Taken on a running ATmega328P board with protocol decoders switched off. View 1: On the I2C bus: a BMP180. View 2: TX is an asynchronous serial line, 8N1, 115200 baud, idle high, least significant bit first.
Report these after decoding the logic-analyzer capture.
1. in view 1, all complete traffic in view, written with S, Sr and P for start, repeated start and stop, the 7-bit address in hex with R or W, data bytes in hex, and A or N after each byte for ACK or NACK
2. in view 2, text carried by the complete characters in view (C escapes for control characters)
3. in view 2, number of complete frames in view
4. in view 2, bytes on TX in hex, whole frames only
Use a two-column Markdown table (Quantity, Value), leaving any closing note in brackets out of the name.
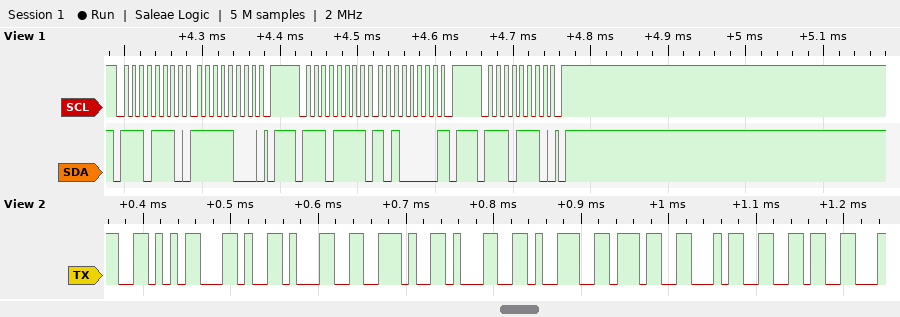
| Quantity | Value |
|---|---|
| in view 1, all complete traffic in view, written with S, Sr and P for start, repeated start and stop, the 7-bit address in hex with R or W, data bytes in hex, and A or N after each byte for ACK or NACK | S 77W A F8 A P S 77R A A0 N P S 77W A P |
| in view 2, text carried by the complete characters in view | "V,1.19746" |
| in view 2, number of complete frames in view | 9 |
| in view 2, bytes on TX in hex, whole frames only | 56 2C 31 2E 31 39 37 34 36 |
